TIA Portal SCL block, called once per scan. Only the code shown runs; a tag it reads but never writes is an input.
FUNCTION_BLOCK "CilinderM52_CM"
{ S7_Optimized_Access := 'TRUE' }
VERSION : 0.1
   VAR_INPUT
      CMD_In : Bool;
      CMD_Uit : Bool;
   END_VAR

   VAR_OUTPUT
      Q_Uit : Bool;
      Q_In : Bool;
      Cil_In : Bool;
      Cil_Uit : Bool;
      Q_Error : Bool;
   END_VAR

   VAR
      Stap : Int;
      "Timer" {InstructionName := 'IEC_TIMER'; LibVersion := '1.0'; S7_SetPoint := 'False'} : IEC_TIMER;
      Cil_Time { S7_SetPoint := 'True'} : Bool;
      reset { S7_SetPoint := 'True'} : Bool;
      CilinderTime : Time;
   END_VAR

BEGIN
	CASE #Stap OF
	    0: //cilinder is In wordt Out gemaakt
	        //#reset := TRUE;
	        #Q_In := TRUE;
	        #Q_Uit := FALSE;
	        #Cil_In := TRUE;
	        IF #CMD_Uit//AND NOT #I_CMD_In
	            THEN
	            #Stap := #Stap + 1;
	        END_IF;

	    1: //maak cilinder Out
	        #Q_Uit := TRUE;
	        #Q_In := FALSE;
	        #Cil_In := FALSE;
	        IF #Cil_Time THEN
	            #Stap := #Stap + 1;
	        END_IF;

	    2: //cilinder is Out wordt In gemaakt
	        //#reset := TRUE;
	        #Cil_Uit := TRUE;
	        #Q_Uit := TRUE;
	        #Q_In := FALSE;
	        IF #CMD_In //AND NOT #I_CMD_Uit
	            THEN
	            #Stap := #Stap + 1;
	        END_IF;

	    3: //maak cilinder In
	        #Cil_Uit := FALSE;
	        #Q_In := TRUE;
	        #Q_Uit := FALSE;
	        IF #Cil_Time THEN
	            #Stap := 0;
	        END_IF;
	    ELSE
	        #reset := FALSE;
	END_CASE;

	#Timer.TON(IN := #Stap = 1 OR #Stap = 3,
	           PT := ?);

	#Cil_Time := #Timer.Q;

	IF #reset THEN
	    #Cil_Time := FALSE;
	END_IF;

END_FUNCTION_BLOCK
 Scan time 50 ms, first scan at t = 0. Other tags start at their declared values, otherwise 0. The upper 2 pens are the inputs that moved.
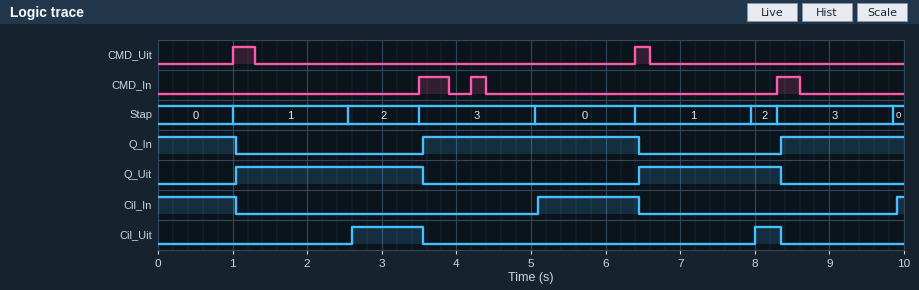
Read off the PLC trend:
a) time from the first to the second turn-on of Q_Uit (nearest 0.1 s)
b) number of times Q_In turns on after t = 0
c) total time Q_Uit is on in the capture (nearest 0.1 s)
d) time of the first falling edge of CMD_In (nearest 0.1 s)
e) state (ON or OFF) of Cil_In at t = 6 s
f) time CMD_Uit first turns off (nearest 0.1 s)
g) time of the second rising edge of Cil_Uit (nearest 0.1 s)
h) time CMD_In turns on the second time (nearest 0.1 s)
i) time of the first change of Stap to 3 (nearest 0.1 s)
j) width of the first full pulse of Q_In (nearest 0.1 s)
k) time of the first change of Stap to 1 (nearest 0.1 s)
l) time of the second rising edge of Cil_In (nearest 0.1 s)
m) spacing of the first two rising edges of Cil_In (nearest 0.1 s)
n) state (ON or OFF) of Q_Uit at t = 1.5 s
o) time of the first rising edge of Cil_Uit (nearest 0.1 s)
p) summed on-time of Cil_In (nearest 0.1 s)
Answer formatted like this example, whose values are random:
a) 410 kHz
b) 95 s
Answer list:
a) 5.4 s
b) 2
c) 4.4 s
d) 3.9 s
e) ON
f) 1.3 s
g) 8.0 s
h) 4.2 s
i) 3.5 s
j) 2.9 s
k) 1.0 s
l) 9.9 s
m) 4.8 s
n) ON
o) 2.6 s
p) 2.5 s
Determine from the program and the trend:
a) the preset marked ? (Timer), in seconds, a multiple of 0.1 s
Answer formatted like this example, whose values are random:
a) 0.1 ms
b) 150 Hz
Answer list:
a) 1.5 s
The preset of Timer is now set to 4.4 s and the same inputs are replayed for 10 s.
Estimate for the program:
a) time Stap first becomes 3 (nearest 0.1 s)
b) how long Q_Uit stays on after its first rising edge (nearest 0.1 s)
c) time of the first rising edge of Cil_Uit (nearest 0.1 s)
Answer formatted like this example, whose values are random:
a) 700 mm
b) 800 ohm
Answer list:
a) 8.3 s
b) 7.3 s
c) 5.5 s
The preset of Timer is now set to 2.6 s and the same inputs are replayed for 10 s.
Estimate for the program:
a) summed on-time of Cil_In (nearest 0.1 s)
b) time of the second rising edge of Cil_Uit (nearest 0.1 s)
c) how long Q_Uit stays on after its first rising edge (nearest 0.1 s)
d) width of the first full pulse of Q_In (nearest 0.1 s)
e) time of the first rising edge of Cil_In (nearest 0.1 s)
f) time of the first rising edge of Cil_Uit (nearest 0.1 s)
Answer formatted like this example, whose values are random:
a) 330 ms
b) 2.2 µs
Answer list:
a) 1.1 s
b) 9.1 s
c) 2.7 s
d) 2.7 s
e) 6.4 s
f) 3.7 s
